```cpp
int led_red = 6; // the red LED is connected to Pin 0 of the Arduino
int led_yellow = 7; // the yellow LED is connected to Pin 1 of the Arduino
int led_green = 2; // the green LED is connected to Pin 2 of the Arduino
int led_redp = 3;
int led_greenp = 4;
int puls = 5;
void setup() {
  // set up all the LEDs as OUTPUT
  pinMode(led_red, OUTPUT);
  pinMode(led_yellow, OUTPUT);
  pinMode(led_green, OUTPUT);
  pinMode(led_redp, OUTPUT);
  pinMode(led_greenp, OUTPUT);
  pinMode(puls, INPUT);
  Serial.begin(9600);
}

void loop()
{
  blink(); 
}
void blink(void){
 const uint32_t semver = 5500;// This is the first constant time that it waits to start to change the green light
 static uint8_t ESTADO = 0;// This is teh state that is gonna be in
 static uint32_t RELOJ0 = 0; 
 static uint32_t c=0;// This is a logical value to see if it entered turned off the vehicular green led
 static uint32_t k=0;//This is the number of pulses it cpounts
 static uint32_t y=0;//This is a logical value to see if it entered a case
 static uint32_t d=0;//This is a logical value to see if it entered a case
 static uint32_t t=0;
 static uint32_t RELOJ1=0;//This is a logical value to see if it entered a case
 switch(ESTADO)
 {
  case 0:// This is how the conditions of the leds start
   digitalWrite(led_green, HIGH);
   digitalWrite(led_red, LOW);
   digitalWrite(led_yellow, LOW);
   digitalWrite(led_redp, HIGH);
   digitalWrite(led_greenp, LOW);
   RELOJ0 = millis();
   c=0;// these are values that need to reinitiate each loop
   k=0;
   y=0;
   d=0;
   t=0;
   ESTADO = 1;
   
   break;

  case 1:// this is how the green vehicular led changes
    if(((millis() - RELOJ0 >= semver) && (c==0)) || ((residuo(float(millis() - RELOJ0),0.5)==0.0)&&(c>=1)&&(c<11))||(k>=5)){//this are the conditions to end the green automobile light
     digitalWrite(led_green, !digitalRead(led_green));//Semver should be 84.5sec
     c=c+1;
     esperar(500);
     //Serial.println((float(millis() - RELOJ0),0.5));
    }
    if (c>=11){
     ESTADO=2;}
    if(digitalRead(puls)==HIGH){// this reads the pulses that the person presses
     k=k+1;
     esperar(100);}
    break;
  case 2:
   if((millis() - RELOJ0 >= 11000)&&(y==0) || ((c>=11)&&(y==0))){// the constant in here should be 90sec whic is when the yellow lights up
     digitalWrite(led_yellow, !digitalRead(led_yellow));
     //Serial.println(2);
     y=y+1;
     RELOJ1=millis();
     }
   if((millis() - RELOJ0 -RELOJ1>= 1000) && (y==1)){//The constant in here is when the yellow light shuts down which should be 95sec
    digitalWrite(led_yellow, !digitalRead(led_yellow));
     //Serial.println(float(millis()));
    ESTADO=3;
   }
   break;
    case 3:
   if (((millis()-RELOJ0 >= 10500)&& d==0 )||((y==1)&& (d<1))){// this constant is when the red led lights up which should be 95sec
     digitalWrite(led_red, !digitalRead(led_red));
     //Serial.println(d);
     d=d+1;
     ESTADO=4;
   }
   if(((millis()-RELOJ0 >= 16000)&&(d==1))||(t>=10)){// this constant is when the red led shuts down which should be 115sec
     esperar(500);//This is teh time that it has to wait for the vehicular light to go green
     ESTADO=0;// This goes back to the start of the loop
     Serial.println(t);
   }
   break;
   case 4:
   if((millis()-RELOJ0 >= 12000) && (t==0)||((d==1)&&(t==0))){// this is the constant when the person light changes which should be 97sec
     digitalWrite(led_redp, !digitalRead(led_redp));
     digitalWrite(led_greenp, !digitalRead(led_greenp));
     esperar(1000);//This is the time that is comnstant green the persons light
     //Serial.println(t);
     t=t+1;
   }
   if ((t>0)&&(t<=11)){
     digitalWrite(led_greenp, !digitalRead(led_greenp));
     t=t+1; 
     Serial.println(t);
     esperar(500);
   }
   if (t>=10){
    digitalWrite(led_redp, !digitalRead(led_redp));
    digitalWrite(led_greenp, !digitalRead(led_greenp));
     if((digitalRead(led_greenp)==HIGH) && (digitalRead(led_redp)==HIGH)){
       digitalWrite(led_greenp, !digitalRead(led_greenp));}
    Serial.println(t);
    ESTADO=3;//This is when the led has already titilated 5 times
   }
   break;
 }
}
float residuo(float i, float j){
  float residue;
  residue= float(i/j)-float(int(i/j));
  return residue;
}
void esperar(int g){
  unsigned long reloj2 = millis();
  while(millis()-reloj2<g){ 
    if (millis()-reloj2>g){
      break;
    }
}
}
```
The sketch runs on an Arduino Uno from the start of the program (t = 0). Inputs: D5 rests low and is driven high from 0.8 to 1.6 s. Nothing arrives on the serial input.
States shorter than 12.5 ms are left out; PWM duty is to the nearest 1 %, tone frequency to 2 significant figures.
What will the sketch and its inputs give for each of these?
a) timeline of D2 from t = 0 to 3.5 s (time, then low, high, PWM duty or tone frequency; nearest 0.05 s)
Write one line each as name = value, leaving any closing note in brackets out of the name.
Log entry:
timeline of D2 from t = 0 to 3.5 s = 0 s high; 1.3 s low; 1.8 s high; 2.3 s low; 2.8 s high; 3.3 s low
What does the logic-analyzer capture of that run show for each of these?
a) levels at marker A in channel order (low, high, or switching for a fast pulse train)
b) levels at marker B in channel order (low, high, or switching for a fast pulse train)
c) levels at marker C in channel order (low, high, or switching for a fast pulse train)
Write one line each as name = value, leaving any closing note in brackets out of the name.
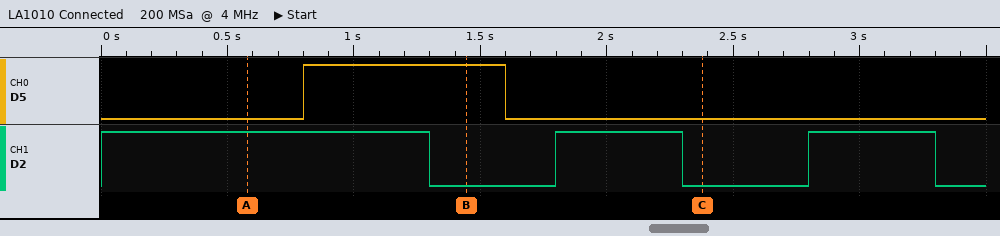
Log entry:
levels at marker A in channel order = D5 low, D2 high
levels at marker B in channel order = D5 high, D2 low
levels at marker C in channel order = D5 low, D2 low
